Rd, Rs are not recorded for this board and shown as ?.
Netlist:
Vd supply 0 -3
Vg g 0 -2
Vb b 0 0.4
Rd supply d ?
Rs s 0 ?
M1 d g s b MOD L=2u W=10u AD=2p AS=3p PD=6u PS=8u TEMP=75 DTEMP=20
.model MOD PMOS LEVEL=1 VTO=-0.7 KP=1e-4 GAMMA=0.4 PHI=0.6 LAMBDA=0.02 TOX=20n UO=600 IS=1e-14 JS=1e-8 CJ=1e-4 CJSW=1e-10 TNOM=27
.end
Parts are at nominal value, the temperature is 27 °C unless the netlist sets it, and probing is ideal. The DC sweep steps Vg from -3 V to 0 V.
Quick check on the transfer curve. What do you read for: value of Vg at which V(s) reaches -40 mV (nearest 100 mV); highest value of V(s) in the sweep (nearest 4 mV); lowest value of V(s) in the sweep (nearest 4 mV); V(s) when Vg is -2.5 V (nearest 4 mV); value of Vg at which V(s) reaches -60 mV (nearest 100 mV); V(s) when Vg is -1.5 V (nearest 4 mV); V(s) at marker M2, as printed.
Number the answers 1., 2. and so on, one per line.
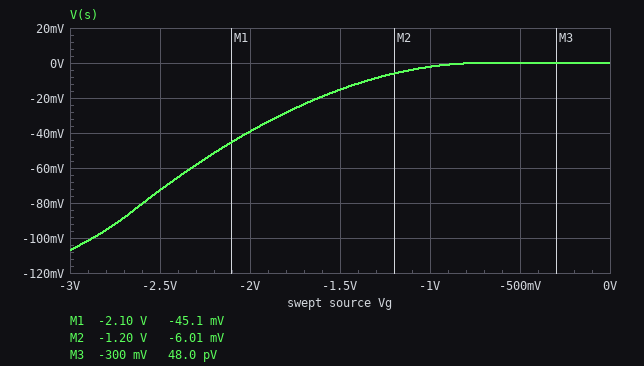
1. -2.0 V
2. 0 V
3. -108 mV
4. -72 mV
5. -2.3 V
6. -16 mV
7. -6.01 mV
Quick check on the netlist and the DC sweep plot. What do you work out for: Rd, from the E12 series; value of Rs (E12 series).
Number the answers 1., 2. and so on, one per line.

1. 1.5 kΩ
2. 120 Ω
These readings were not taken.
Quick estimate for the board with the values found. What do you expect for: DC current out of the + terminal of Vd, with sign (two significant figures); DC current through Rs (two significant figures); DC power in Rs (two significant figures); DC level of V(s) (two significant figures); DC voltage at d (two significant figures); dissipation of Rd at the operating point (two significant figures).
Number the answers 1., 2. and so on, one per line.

1. -330 µA
2. 330 µA
3. 13 µW
4. -39 mV
5. -2.5 V
6. 160 µW
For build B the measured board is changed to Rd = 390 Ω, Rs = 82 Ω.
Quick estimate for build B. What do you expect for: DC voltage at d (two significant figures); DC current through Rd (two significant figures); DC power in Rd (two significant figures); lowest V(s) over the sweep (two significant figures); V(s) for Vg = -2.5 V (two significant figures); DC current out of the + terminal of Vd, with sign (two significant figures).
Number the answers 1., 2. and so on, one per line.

1. -2.9 V
2. 340 µA
3. 44 µW
4. -83 mV
5. -52 mV
6. -340 µA
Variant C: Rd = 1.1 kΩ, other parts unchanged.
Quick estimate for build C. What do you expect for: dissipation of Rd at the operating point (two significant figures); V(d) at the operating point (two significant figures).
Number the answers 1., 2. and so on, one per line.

1. 120 µW
2. -2.6 V
